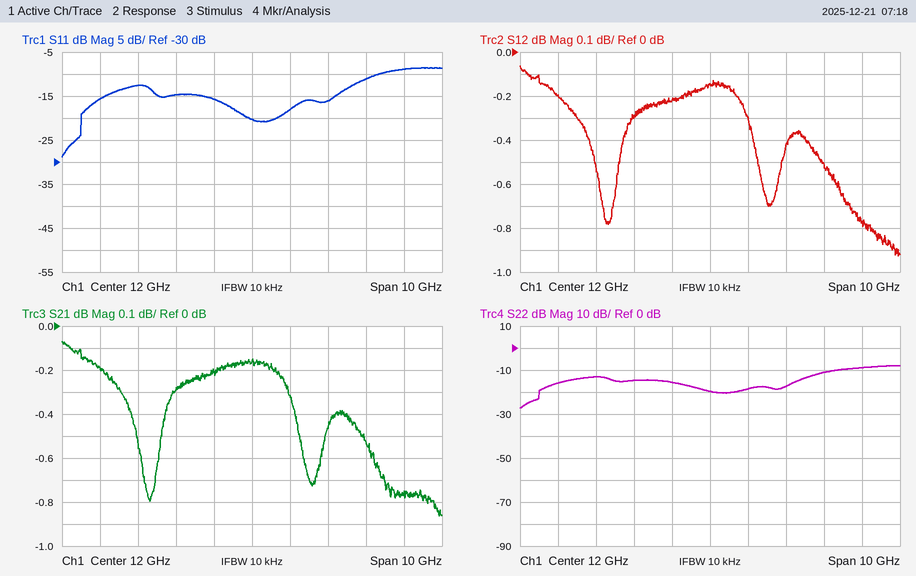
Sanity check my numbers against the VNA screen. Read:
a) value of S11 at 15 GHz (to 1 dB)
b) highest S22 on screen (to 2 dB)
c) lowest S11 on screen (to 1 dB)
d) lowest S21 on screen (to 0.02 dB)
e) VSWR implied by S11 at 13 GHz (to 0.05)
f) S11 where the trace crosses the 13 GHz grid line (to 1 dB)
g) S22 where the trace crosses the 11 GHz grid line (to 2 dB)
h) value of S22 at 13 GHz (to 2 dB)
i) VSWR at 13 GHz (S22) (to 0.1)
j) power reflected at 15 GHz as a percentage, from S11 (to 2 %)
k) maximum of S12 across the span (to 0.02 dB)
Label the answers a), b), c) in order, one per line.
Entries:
a) -11 dB
b) -8 dB
c) -29 dB
d) -0.86 dB
e) 1.30
f) -18 dB
g) -16 dB
h) -18 dB
i) 1.3
j) 8 %
k) -0.06 dB
